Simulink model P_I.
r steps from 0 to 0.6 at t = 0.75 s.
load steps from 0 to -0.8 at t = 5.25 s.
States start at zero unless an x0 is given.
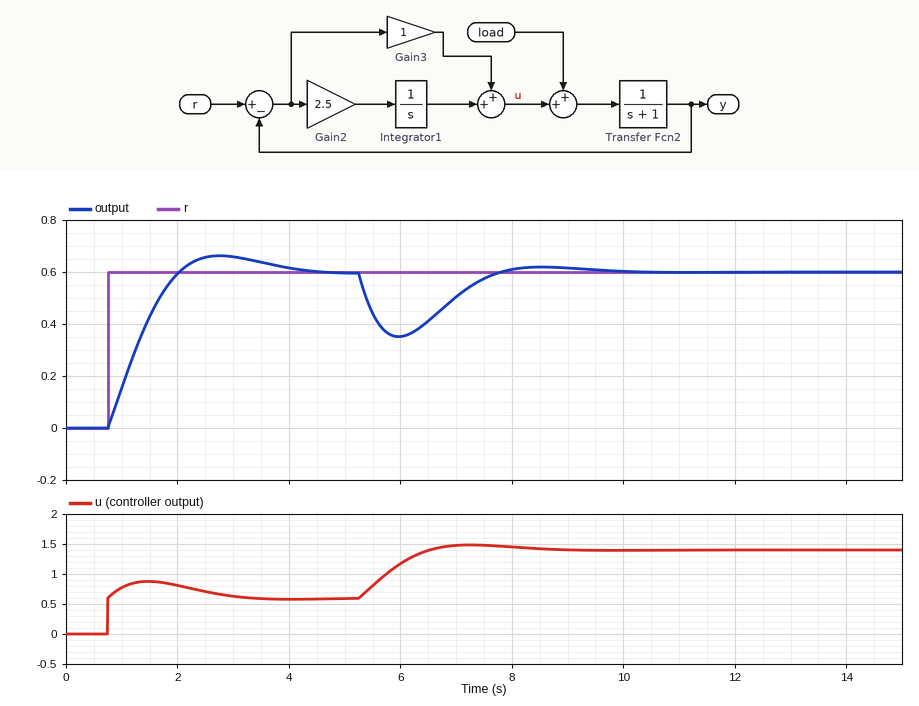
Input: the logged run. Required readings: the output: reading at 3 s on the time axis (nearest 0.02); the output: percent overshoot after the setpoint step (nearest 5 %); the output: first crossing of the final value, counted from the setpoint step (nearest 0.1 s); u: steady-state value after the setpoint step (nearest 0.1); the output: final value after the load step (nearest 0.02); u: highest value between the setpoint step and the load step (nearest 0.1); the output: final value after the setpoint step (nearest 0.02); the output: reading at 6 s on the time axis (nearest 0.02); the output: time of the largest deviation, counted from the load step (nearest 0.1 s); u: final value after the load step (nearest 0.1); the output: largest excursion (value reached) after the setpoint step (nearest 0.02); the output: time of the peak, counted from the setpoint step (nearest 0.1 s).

0.66
10 %
1.3 s
0.6
0.60
0.9
0.60
0.36
0.7 s
1.4
0.66
2.0 s
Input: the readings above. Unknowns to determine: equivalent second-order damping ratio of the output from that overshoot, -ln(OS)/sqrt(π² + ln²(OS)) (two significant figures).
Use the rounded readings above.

0.59
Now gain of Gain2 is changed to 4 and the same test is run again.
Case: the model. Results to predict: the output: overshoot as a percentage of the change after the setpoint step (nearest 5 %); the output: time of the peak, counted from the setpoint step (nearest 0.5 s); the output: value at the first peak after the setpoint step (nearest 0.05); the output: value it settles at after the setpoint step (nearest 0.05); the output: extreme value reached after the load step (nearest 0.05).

20 %
1.5 s
0.70
0.60
0.40
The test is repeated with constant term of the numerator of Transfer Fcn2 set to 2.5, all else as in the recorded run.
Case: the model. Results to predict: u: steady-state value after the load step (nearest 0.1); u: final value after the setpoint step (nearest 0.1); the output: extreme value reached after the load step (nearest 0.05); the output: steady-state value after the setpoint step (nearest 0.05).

1.0
0.2
0.25
0.60
